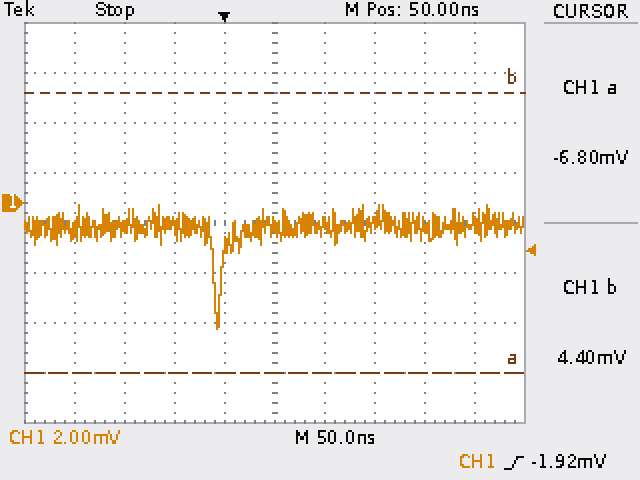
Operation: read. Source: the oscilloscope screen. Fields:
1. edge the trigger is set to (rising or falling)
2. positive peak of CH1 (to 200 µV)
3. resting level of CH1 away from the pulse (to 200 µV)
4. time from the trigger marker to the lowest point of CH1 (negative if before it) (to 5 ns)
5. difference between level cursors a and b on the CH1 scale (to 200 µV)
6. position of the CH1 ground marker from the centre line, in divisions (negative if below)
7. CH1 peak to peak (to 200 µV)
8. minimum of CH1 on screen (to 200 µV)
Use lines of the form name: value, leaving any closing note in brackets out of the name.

edge the trigger is set to: rising
positive peak of CH1: 0.0 mV
resting level of CH1 away from the pulse: -1.0 mV
time from the trigger marker to the lowest point of CH1 (negative if before it): -5 ns
difference between level cursors a and b on the CH1 scale: 11.2 mV
position of the CH1 ground marker from the centre line, in divisions: +0.4 div
CH1 peak to peak: 5.0 mV
minimum of CH1 on screen: -5.0 mV
